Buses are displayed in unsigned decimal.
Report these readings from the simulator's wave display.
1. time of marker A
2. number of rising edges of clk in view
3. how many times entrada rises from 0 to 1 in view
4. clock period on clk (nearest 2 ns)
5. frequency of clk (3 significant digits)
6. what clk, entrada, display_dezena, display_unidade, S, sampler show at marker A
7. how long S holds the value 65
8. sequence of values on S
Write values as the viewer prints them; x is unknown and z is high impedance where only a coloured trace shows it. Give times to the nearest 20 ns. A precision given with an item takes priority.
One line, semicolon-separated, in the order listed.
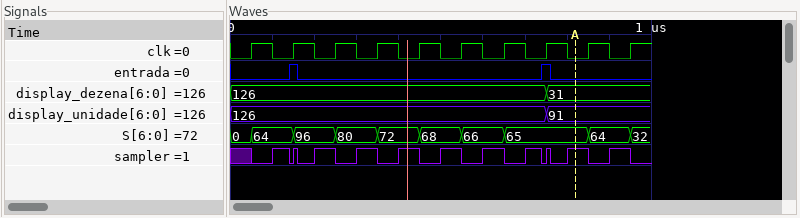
820 ns; 10; 2; 100 ns; 10.0 MHz; clk=0, entrada=0, display_dezena=31, display_unidade=91, S=65, sampler=1; 200 ns; 0, 64, 96, 80, 72, 68, 66, 65, 64, 32
